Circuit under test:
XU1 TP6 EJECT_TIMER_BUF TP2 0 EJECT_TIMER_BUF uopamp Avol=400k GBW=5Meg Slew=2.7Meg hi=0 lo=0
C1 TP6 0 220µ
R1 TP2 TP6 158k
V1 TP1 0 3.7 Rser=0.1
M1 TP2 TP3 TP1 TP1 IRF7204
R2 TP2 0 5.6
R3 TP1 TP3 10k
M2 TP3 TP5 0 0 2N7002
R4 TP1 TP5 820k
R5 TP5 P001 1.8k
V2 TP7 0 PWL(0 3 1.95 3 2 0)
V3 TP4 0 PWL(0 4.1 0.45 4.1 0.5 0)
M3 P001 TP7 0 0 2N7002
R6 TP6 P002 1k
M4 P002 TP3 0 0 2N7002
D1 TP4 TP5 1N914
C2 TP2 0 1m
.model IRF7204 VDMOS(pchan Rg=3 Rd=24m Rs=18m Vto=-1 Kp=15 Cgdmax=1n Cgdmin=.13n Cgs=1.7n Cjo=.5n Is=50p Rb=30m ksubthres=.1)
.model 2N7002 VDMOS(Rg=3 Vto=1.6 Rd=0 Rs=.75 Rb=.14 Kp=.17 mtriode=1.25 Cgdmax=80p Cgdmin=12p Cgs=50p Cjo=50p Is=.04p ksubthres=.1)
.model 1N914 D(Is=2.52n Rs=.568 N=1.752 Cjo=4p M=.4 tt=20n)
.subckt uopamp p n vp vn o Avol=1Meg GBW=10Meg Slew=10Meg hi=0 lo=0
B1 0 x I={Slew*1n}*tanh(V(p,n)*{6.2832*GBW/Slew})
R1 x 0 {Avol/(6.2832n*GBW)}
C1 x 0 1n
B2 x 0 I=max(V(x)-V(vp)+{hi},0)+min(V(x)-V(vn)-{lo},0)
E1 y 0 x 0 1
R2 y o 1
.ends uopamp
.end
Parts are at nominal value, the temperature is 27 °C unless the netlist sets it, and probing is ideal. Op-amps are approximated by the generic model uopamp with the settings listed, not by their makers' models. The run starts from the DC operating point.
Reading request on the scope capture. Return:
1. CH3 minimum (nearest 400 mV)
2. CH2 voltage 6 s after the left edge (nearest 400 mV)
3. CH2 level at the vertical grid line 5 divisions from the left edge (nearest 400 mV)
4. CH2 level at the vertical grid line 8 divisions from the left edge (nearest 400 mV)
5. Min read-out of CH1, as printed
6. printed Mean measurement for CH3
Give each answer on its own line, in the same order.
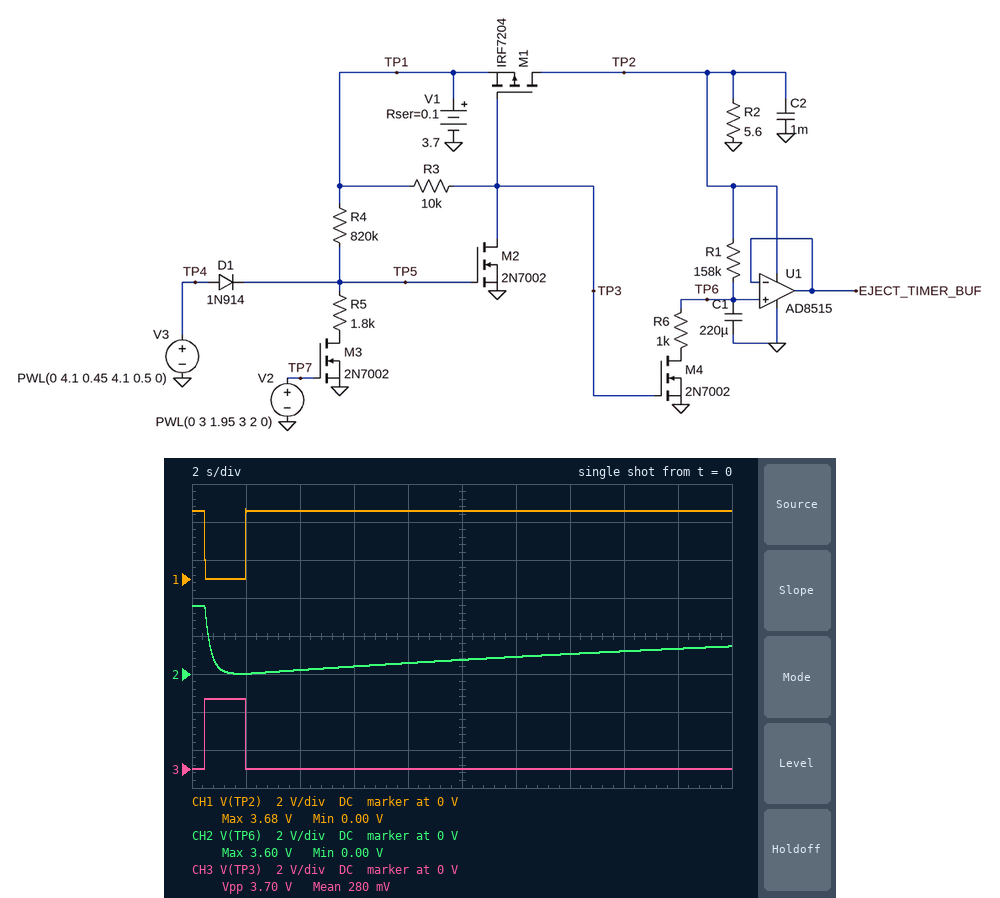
0 V
400 mV
800 mV
1.2 V
0.00 V
280 mV
